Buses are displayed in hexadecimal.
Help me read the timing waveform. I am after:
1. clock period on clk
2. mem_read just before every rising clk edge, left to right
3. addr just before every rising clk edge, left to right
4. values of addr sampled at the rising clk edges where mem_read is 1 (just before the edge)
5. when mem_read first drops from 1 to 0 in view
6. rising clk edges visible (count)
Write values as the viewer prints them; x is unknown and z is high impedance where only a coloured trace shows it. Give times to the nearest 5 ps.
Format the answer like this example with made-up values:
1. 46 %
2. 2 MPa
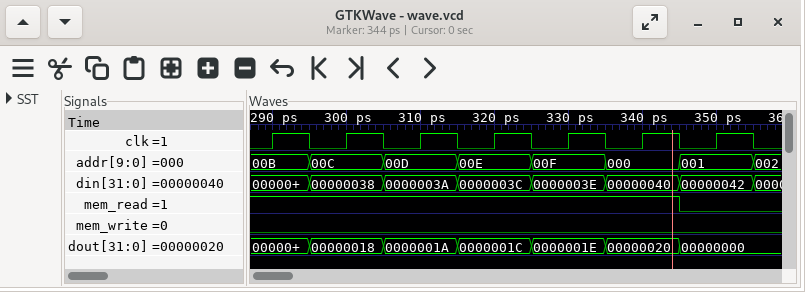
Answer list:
1. 10 ps
2. 1 1 1 1 1 1 0
3. 00B, 00C, 00D, 00E, 00F, 000, 001
4. 00B, 00C, 00D, 00E, 00F, 000
5. 345 ps
6. 7
